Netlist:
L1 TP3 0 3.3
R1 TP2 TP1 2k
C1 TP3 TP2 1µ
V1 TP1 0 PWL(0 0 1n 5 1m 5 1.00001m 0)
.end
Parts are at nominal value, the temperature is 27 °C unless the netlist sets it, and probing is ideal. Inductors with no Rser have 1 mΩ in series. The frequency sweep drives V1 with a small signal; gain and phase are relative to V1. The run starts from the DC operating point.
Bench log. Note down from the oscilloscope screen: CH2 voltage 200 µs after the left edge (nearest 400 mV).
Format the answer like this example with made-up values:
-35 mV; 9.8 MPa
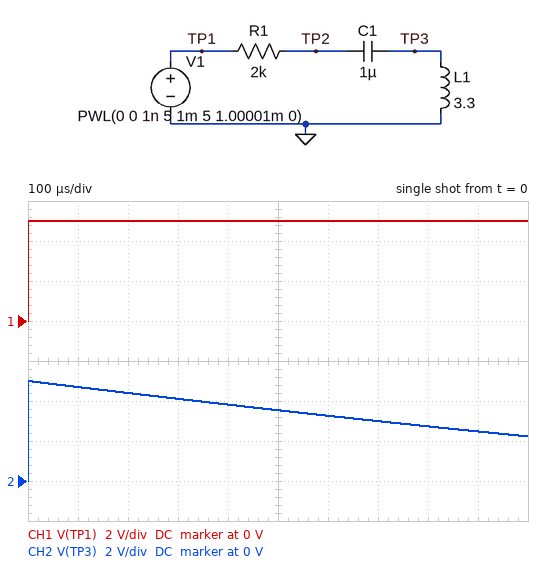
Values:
4.4 V
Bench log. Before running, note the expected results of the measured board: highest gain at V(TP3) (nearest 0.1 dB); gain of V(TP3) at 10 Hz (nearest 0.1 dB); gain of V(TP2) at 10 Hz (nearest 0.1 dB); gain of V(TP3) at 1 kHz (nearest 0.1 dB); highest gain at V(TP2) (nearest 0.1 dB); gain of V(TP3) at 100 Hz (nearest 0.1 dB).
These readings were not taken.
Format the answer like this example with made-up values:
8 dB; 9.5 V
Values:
0.7 dB; -37.7 dB; -0.1 dB; 0 dB; 0 dB; 0.1 dB
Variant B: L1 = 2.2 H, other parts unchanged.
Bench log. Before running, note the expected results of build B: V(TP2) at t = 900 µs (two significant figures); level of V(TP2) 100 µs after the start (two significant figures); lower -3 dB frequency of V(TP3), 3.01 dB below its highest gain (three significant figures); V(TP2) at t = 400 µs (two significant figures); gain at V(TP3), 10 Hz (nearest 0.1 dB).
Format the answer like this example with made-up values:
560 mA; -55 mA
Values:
2.4 V; 4.6 V; 103 Hz; 3.5 V; -41.2 dB
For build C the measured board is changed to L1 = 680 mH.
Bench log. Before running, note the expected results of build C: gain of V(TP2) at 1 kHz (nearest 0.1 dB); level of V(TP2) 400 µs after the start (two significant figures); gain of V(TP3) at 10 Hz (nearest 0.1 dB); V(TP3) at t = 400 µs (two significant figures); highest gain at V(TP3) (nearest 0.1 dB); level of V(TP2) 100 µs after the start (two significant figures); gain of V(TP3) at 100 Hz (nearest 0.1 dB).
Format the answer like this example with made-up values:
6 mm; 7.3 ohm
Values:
-0.9 dB; 1.7 V; -51.5 dB; 1.3 V; 0 dB; 3.7 V; -14.7 dB
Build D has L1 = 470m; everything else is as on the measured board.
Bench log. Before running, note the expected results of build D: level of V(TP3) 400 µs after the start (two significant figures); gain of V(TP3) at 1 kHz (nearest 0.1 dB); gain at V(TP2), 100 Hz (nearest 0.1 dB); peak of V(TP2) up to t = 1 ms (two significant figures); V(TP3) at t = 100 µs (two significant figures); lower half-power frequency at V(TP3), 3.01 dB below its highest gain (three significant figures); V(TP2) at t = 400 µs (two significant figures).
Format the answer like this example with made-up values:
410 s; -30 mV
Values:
620 mV; -1.3 dB; -5.3 dB; 5.0 V; 3.2 V; 599 Hz; 1.1 V
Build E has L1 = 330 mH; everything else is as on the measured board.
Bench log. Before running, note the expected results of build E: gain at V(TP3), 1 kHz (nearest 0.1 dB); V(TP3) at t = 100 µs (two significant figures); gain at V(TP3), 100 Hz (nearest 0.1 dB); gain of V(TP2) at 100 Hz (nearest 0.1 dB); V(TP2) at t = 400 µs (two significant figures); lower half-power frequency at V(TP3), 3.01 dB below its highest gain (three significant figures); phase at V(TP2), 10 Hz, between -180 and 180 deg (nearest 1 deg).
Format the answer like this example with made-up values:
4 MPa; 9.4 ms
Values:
-2.5 dB; 2.7 V; -21.4 dB; -4.9 dB; 770 mV; 886 Hz; -7 deg
